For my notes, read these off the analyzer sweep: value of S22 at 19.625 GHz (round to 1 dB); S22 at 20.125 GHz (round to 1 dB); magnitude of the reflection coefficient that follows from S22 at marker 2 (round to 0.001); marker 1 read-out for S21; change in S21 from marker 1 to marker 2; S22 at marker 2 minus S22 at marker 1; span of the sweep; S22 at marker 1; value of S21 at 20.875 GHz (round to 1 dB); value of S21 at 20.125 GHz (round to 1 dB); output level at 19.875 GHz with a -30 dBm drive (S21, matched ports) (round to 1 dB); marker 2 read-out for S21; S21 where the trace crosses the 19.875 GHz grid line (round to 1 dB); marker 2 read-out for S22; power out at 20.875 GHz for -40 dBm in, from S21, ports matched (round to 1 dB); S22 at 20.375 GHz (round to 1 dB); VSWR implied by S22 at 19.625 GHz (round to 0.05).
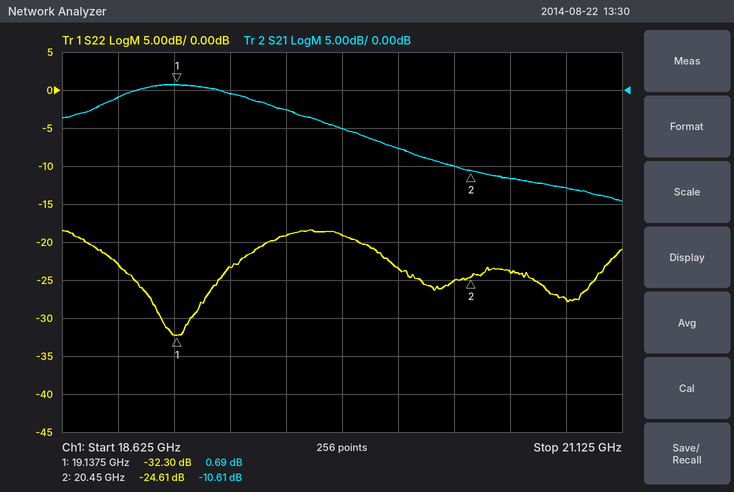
-19 dB
-23 dB
0.059
0.69 dB
-11.30 dB
7.69 dB
2.5 GHz
-32.30 dB
-13 dB
-8 dB
-35 dBm
-10.61 dB
-5 dB
-24.61 dB
-53 dBm
-25 dB
1.25
